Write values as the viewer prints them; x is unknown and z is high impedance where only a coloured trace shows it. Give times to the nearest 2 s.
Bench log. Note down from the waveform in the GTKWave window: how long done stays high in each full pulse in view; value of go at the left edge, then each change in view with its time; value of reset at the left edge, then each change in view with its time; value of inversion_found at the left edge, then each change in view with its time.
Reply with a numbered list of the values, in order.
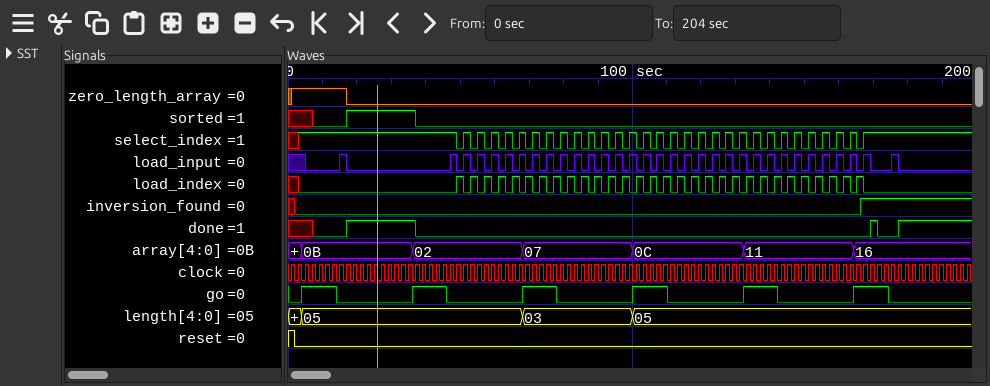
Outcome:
1. 20 s, 2 s
2. 0, 1 at 4 s, 0 at 14 s, 1 at 36 s, 0 at 46 s, 1 at 68 s, 0 at 78 s, 1 at 100 s, 0 at 110 s, 1 at 132 s, 0 at 142 s, 1 at 164 s, 0 at 174 s
3. 1, 0 at 2 s
4. x, 0 at 2 s, 1 at 166 s
